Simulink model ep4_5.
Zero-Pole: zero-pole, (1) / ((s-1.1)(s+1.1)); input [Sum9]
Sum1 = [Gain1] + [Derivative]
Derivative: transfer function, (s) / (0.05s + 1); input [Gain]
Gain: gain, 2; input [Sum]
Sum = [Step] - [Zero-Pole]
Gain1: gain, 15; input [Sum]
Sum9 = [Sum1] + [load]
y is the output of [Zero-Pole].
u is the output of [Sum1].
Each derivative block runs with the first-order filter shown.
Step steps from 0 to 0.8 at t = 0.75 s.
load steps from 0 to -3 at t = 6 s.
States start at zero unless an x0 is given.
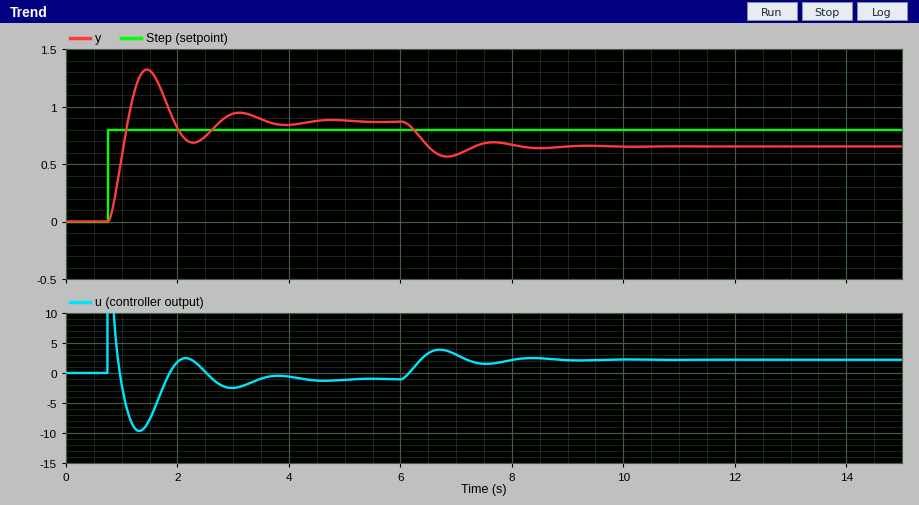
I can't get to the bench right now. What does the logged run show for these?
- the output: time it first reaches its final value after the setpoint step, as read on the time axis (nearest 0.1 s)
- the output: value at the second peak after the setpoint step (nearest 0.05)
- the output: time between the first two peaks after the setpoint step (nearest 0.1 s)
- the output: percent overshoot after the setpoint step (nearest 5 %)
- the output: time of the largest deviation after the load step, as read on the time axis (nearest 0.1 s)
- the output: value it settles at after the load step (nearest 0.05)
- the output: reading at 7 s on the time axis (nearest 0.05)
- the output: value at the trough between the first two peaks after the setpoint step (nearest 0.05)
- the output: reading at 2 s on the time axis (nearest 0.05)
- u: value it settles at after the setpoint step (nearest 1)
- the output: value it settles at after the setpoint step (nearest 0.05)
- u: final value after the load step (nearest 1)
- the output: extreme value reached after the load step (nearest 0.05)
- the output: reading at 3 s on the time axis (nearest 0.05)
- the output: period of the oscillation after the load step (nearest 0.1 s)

1.1 s
0.95
1.7 s
50 %
6.8 s
0.65
0.60
0.70
0.80
-1
0.85
2
0.55
0.95
1.7 s
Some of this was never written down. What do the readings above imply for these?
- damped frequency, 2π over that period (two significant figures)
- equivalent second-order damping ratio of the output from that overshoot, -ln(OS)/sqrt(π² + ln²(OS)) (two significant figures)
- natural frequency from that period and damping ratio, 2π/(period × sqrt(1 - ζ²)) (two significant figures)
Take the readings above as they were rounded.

3.7 rad/s
0.22
3.8 rad/s
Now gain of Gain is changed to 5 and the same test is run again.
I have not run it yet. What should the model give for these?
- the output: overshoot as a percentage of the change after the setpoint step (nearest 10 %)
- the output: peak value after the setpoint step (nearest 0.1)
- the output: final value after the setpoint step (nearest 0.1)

20 %
1.1
0.9
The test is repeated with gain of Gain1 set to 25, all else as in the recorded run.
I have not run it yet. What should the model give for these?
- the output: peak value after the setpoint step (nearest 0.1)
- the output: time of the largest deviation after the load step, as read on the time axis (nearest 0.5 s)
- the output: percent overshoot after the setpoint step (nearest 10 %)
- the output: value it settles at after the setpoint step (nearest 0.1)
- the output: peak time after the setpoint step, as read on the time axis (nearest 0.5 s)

1.4
6.5 s
60 %
0.8
1.5 s
